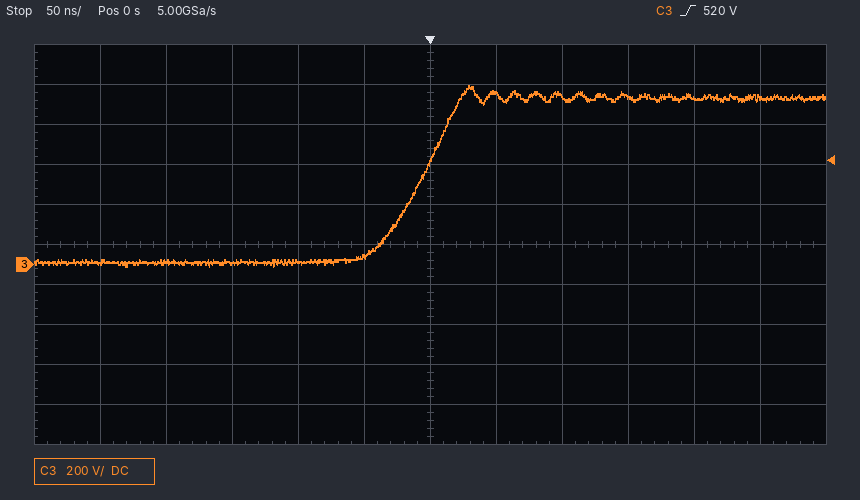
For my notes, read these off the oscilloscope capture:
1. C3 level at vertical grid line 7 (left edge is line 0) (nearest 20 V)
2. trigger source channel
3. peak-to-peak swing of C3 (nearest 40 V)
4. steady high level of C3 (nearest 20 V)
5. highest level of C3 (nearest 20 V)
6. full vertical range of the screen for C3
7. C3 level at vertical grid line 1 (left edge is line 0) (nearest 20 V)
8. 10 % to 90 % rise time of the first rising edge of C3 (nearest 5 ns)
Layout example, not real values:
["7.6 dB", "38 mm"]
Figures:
["860 V", "C3", "920 V", "840 V", "900 V", "2 kV", "20 V", "55 ns"]
